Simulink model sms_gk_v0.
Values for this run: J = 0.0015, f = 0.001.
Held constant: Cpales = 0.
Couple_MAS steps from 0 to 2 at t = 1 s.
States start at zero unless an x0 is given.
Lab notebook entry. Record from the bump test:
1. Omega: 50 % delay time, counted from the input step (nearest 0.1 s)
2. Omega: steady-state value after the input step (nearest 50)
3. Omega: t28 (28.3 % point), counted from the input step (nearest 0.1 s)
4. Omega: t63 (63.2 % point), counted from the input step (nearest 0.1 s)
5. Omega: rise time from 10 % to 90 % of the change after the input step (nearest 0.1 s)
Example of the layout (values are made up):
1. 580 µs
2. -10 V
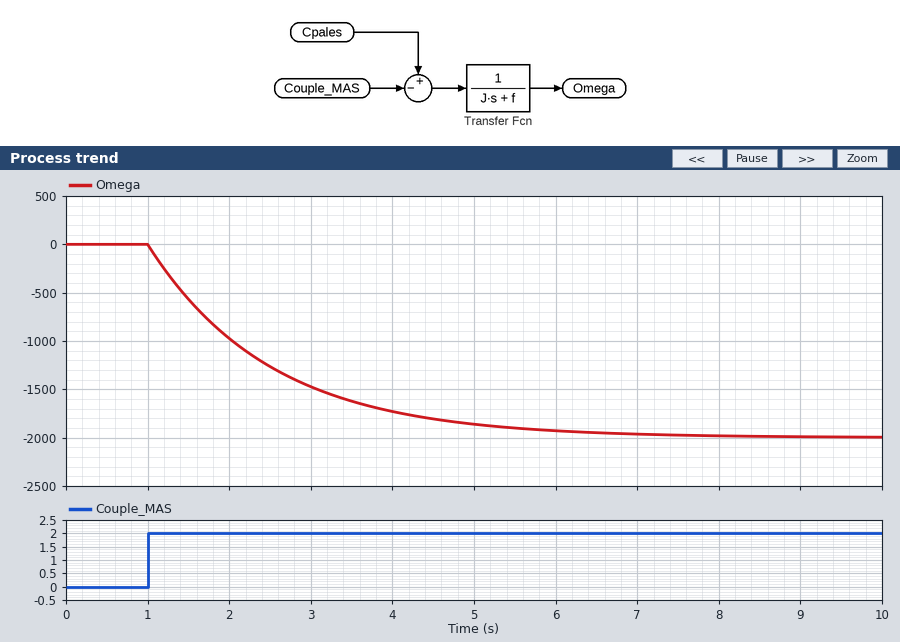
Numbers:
1. 1.0 s
2. -2000
3. 0.5 s
4. 1.5 s
5. 3.3 s
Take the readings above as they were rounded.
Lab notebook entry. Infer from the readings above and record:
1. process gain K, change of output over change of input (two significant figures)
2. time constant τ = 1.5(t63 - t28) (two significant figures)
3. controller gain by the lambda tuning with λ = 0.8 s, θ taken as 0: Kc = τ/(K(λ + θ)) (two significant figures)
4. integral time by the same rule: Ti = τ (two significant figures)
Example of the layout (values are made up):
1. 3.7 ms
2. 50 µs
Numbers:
1. -1000
2. 1.5 s
3. -0.0019
4. 1.5 s
